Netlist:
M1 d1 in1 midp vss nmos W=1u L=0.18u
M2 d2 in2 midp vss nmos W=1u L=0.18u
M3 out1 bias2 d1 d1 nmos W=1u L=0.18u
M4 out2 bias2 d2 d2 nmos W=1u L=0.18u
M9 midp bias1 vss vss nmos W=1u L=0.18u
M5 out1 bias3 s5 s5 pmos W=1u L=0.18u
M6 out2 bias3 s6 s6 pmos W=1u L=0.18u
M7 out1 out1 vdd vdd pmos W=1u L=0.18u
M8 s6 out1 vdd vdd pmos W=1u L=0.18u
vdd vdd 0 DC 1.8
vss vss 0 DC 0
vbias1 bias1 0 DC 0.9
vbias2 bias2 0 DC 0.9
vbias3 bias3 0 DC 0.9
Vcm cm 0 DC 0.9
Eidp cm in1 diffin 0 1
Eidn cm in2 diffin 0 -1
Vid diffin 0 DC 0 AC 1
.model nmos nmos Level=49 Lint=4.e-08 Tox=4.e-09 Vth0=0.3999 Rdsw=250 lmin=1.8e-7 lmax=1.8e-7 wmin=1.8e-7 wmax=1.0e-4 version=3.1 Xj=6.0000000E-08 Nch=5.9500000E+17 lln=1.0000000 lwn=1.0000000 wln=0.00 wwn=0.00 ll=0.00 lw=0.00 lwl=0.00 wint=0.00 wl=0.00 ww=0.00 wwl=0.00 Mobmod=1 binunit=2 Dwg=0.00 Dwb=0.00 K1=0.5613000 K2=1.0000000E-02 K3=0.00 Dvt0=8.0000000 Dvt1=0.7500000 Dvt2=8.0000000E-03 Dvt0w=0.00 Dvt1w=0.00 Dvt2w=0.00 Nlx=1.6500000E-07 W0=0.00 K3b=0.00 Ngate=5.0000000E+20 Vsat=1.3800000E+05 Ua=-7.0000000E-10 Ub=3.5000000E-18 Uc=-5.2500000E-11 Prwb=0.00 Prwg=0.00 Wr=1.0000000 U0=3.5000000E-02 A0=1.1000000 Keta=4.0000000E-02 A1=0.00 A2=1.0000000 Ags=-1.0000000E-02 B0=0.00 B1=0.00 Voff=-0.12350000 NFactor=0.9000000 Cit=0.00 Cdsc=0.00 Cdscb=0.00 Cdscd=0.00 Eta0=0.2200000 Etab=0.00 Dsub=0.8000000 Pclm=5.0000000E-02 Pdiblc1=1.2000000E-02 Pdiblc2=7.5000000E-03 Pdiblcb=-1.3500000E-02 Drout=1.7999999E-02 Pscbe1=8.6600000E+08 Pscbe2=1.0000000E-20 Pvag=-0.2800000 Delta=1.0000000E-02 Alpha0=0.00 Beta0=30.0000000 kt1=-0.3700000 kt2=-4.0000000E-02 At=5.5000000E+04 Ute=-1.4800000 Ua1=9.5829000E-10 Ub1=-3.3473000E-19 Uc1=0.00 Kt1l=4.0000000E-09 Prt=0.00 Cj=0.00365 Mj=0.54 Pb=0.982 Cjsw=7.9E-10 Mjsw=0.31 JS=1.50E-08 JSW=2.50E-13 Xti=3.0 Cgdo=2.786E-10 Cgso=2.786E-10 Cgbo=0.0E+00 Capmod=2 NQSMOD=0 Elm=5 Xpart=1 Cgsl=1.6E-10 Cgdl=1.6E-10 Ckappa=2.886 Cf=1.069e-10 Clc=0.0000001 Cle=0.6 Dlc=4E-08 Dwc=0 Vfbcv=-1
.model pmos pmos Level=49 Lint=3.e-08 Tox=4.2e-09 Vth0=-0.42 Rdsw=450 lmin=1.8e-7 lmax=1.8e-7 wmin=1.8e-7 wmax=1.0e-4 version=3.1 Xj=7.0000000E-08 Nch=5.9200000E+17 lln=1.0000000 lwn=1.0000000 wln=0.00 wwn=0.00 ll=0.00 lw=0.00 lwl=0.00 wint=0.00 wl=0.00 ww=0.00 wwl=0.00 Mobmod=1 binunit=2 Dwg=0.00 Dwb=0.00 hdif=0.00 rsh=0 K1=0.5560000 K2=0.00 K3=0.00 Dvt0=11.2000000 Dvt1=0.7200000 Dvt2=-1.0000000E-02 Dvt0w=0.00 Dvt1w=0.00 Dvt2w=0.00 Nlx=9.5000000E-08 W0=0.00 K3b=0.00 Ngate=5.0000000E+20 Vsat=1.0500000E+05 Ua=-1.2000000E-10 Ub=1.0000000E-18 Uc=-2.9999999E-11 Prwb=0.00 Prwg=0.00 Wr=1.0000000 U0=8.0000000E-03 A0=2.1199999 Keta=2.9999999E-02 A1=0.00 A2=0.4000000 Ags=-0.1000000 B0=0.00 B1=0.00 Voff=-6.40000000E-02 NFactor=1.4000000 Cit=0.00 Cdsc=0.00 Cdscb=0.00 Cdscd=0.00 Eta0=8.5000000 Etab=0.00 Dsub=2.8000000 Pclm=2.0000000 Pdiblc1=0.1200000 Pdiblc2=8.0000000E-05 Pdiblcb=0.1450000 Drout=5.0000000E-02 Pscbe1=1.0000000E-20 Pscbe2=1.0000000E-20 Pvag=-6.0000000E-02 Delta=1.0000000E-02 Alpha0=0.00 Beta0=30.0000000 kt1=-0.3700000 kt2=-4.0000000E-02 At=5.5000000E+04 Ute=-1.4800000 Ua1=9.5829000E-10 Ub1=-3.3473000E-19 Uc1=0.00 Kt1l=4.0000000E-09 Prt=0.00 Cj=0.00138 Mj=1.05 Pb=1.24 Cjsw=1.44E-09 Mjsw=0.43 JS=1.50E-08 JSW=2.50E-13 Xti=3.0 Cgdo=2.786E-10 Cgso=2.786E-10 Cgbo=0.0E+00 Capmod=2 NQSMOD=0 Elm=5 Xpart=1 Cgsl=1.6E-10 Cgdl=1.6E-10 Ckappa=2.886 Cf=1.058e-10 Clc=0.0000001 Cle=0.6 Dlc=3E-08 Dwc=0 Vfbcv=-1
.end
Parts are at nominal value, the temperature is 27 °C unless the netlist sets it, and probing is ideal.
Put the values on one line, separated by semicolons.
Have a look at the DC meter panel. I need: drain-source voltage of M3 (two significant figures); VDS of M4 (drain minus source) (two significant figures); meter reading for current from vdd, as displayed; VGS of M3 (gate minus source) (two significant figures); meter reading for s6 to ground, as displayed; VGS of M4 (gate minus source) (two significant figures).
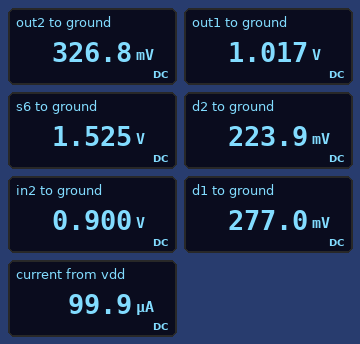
740 mV; 100 mV; 99.9 µA; 620 mV; 1.525 V; 680 mV
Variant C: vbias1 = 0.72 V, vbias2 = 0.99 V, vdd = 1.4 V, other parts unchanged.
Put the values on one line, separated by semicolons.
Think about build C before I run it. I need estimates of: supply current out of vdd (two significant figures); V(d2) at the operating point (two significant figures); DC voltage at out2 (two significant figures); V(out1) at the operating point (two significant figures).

68 µA; 200 mV; 220 mV; 630 mV
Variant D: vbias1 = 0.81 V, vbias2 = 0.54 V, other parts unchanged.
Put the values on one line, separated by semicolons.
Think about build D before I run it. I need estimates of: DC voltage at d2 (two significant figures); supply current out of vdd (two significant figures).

75 mV; 36 µA
